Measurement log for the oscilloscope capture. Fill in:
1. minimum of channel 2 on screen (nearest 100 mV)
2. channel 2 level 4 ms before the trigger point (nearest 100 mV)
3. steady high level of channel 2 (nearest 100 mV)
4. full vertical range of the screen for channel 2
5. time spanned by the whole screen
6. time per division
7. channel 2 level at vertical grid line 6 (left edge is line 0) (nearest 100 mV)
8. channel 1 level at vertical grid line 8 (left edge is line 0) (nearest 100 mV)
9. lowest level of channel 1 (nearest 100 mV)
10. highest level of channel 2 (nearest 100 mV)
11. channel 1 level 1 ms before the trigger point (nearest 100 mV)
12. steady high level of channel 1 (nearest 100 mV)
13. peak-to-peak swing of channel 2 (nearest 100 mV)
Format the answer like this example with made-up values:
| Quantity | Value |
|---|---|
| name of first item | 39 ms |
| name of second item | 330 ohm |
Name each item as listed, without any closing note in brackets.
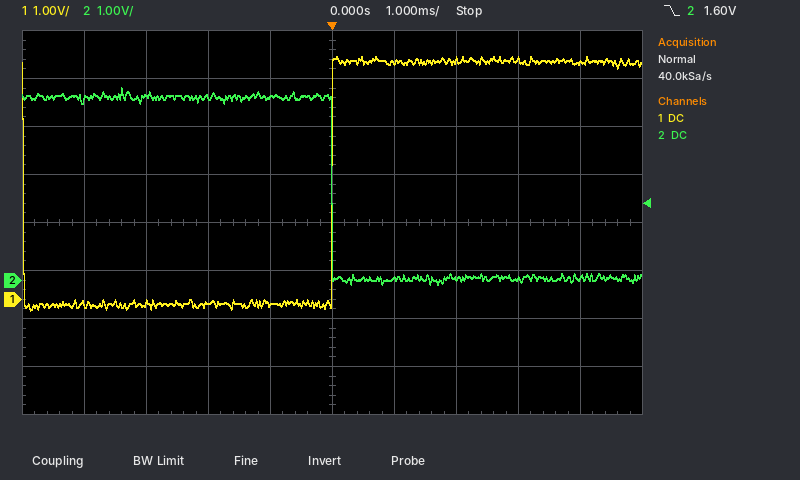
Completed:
| Quantity | Value |
|---|---|
| minimum of channel 2 on screen | -100 mV |
| channel 2 level 4 ms before the trigger point | 3.8 V |
| steady high level of channel 2 | 3.8 V |
| full vertical range of the screen for channel 2 | 8 V |
| time spanned by the whole screen | 10 ms |
| time per division | 1 ms |
| channel 2 level at vertical grid line 6 (left edge is line 0) | 0.0 V |
| channel 1 level at vertical grid line 8 (left edge is line 0) | 5.0 V |
| lowest level of channel 1 | -200 mV |
| highest level of channel 2 | 4.0 V |
| channel 1 level 1 ms before the trigger point | -100 mV |
| steady high level of channel 1 | 5.0 V |
| peak-to-peak swing of channel 2 | 4.1 V |
